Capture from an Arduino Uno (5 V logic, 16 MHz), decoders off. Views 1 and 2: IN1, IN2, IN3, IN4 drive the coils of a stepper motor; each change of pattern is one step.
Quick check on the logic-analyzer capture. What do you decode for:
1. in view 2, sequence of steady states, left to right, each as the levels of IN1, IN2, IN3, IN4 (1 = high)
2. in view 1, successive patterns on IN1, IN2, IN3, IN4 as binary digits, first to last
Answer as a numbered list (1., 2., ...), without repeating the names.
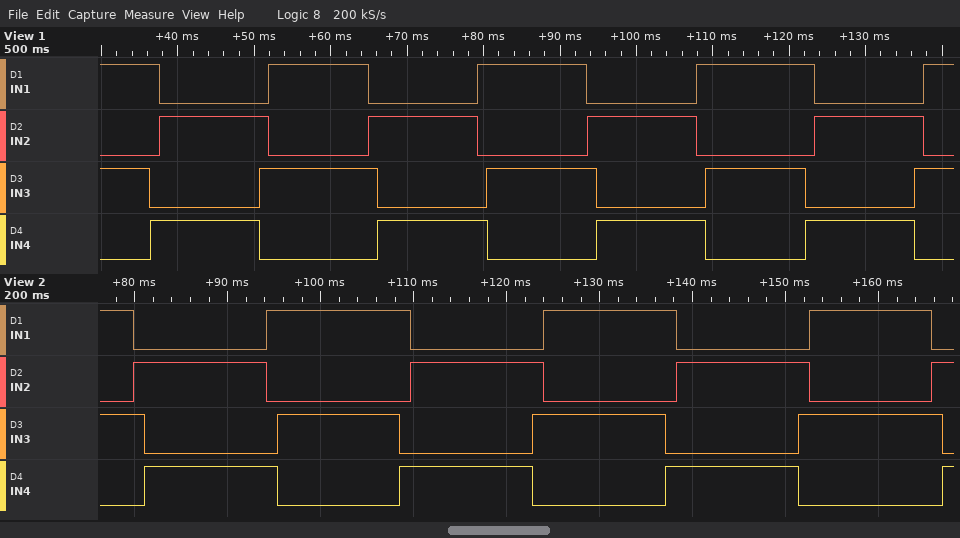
1. 1010 0110 0101 1001 1010 1001 0101 0110 1010 1001 0101 0110 1010 0110 0101
2. 1010 1001 0101 0110 1010 0110 0101 1001 1010 0110 0101 1001 1010 1001 0101 0110 1010
